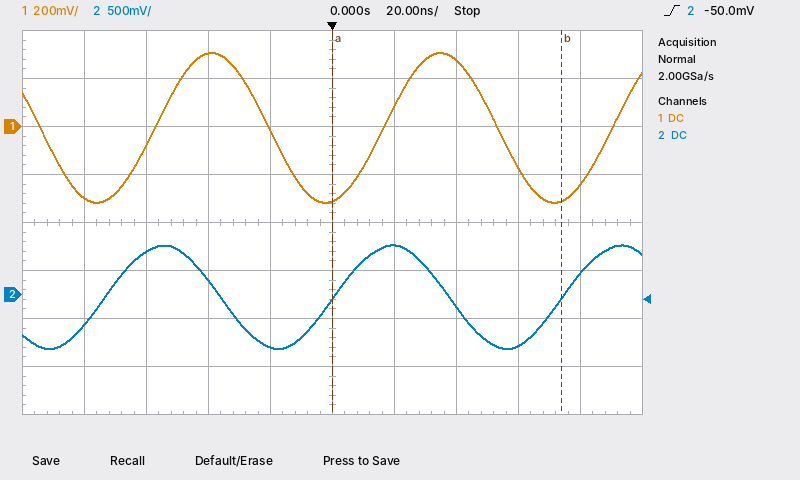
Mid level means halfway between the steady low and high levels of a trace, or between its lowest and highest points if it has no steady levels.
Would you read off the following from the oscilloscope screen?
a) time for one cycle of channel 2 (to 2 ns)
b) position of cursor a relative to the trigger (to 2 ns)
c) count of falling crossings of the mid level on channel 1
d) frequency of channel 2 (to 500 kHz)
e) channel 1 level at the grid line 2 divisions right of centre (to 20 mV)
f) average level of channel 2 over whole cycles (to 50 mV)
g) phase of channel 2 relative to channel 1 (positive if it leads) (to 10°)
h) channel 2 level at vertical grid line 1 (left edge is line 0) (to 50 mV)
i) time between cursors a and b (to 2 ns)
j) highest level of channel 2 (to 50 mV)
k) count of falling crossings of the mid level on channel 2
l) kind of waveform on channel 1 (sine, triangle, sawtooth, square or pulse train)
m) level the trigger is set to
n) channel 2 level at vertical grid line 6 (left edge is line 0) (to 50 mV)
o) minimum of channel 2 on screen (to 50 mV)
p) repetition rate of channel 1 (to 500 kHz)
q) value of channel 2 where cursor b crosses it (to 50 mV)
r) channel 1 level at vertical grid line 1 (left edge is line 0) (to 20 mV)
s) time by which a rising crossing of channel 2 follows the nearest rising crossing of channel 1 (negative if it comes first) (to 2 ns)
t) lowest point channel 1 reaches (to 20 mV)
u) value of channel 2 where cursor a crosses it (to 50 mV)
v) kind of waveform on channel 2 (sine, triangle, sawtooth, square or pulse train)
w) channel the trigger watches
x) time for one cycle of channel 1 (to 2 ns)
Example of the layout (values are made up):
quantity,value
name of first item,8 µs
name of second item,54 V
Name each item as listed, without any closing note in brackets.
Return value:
quantity,value
time for one cycle of channel 2,74 ns
position of cursor a relative to the trigger,0 ns
count of falling crossings of the mid level on channel 1,3
frequency of channel 2,13.5 MHz
channel 1 level at the grid line 2 divisions right of centre,280 mV
average level of channel 2 over whole cycles,0 mV
phase of channel 2 relative to channel 1 (positive if it leads),+80°
channel 2 level at vertical grid line 1 (left edge is line 0),-300 mV
time between cursors a and b,74 ns
highest level of channel 2,500 mV
count of falling crossings of the mid level on channel 2,2
kind of waveform on channel 1,sine
level the trigger is set to,-50.0 mV
channel 2 level at vertical grid line 6 (left edge is line 0),500 mV
minimum of channel 2 on screen,-550 mV
repetition rate of channel 1,13.5 MHz
value of channel 2 where cursor b crosses it,-50 mV
channel 1 level at vertical grid line 1 (left edge is line 0),-300 mV
time by which a rising crossing of channel 2 follows the nearest rising crossing of channel 1 (negative if it comes first),-16 ns
lowest point channel 1 reaches,-320 mV
value of channel 2 where cursor a crosses it,-50 mV
kind of waveform on channel 2,sine
channel the trigger watches,channel 2
time for one cycle of channel 1,74 ns
